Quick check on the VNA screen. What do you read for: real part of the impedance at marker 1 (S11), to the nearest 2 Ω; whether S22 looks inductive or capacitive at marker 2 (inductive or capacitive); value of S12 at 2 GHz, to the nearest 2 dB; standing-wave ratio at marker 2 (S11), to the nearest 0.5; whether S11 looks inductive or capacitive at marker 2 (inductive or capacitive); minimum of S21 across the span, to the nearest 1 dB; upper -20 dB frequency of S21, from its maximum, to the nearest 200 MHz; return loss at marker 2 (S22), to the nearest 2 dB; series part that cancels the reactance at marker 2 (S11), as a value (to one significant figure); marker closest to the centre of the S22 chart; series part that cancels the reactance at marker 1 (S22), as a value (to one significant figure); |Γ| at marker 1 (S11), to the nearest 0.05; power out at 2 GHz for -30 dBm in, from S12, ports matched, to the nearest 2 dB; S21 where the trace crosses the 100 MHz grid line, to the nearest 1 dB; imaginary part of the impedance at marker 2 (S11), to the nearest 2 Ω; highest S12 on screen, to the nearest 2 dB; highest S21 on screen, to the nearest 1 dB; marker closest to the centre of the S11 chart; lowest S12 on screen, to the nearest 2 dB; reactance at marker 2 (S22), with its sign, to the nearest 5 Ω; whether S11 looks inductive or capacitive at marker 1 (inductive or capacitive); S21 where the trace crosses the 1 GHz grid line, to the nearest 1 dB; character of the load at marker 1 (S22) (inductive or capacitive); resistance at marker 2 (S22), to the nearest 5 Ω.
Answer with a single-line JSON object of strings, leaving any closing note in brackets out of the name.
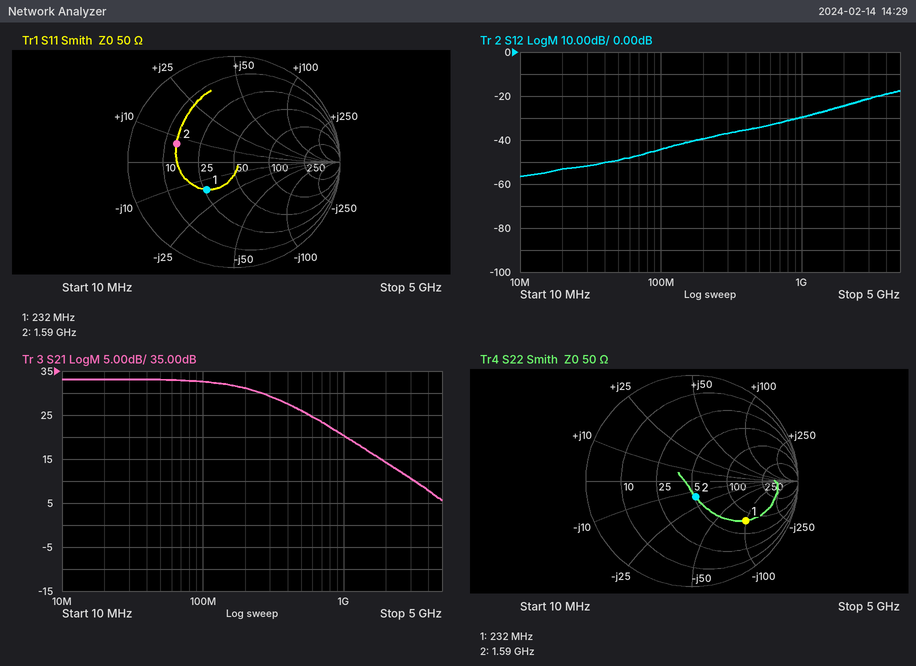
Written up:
{"real part of the impedance at marker 1 (S11), to the nearest 2 Ω": "26 Ω", "whether S22 looks inductive or capacitive at marker 2": "capacitive", "value of S12 at 2 GHz, to the nearest 2 dB": "-24 dB", "standing-wave ratio at marker 2 (S11), to the nearest 0.5": "3.5", "whether S11 looks inductive or capacitive at marker 2": "inductive", "minimum of S21 across the span, to the nearest 1 dB": "6 dB", "upper -20 dB frequency of S21, from its maximum, to the nearest 200 MHz": "2.2 GHz", "return loss at marker 2 (S22), to the nearest 2 dB": "16 dB", "series part that cancels the reactance at marker 2 (S11), as a value": "10 pF", "marker closest to the centre of the S22 chart": "marker 2", "series part that cancels the reactance at marker 1 (S22), as a value": "70 nH", "|Γ| at marker 1 (S11), to the nearest 0.05": "0.35", "power out at 2 GHz for -30 dBm in, from S12, ports matched, to the nearest 2 dB": "-54 dBm", "S21 where the trace crosses the 100 MHz grid line, to the nearest 1 dB": "33 dB", "imaginary part of the impedance at marker 2 (S11), to the nearest 2 Ω": "+8 Ω", "highest S12 on screen, to the nearest 2 dB": "-18 dB", "highest S21 on screen, to the nearest 1 dB": "33 dB", "marker closest to the centre of the S11 chart": "marker 1", "lowest S12 on screen, to the nearest 2 dB": "-56 dB", "reactance at marker 2 (S22), with its sign, to the nearest 5 Ω": "-15 Ω", "whether S11 looks inductive or capacitive at marker 1": "capacitive", "S21 where the trace crosses the 1 GHz grid line, to the nearest 1 dB": "20 dB", "character of the load at marker 1 (S22)": "capacitive", "resistance at marker 2 (S22), to the nearest 5 Ω": "50 Ω"}
